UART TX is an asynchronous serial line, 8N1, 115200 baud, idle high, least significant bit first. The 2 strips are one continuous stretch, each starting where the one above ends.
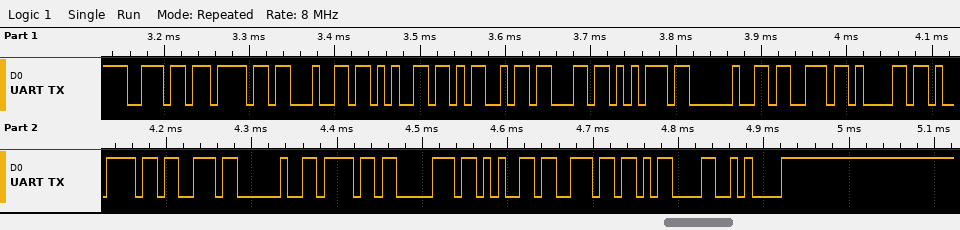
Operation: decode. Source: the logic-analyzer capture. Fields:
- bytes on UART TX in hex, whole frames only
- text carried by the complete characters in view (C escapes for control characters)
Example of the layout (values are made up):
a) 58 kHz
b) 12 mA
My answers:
a) 6E 6F 64 65 4D 63 75 20 73 61 79 73 20 6F 70 65 6E 0D 0A
b) "nodeMcu says open\r\n"
